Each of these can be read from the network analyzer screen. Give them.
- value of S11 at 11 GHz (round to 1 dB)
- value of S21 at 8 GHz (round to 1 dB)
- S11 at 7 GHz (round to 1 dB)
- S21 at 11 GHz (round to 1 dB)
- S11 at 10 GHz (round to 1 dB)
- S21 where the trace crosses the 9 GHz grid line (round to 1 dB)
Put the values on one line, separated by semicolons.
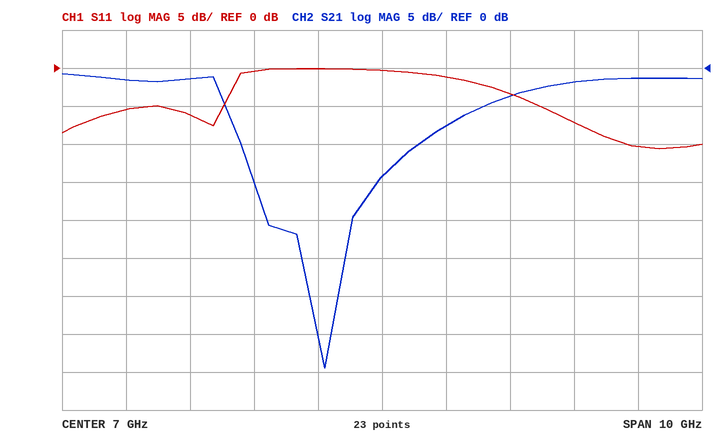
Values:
-10 dB; -8 dB; 0 dB; -1 dB; -7 dB; -4 dB
